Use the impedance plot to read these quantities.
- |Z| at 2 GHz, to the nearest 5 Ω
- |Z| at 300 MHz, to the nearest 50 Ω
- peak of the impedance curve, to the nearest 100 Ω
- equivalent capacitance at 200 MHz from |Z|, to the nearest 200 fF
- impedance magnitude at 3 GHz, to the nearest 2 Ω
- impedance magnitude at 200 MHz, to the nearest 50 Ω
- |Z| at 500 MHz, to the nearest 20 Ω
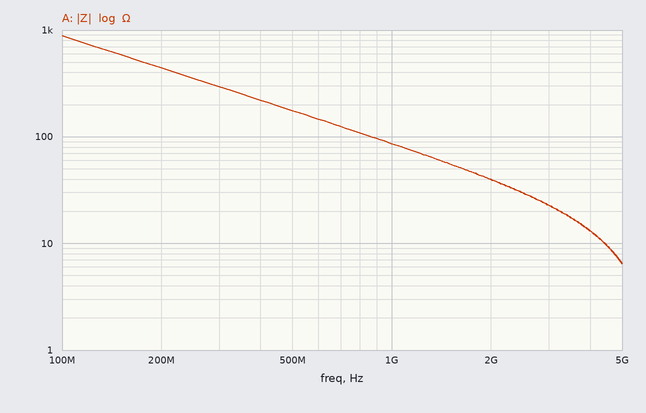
40 Ω
300 Ω
900 Ω
1.8 pF
22 Ω
450 Ω
180 Ω
